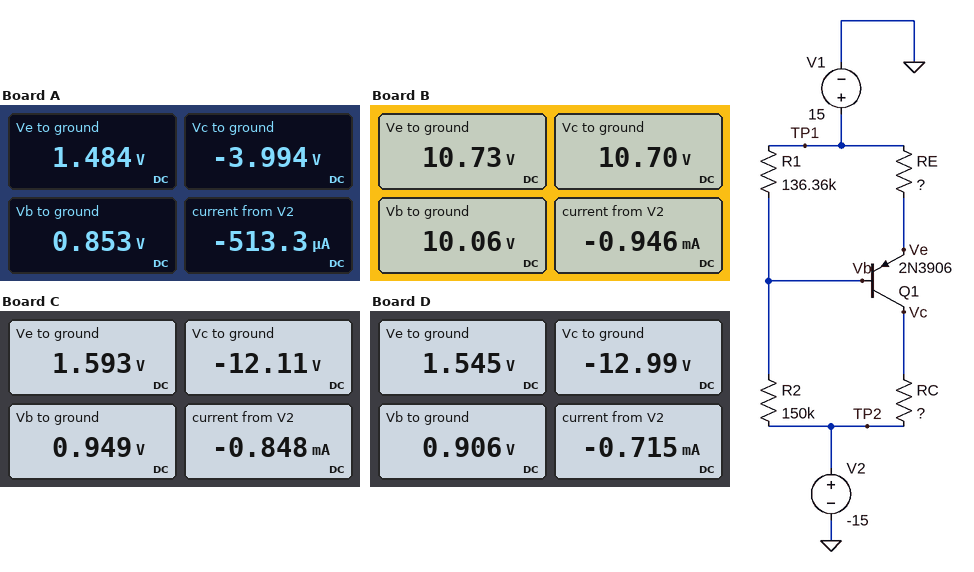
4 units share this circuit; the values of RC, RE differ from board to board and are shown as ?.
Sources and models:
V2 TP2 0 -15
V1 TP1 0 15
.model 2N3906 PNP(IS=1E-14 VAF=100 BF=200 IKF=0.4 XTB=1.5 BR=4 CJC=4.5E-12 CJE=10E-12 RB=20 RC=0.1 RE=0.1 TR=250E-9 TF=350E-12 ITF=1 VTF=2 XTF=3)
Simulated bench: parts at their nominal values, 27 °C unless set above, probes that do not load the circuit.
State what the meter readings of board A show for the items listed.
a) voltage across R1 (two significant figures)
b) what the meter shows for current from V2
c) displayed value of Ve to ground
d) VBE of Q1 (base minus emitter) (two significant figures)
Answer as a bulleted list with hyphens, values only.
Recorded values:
- 14 V
- -513.3 µA
- 1.484 V
- -630 mV
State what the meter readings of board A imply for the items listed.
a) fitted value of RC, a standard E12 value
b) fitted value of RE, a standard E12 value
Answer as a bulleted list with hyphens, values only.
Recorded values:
- 27 kΩ
- 33 kΩ
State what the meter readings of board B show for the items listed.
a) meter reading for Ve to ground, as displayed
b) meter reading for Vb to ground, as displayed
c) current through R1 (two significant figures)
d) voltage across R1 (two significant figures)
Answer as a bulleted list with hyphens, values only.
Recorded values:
- 10.73 V
- 10.06 V
- 36 µA
- 4.9 V
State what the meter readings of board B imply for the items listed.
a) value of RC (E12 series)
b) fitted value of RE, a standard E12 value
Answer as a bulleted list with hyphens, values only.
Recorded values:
- 33 kΩ
- 4.7 kΩ
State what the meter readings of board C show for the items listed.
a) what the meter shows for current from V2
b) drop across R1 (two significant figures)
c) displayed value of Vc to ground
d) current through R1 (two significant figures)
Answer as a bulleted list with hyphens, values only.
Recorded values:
- -0.848 mA
- 14 V
- -12.11 V
- 100 µA
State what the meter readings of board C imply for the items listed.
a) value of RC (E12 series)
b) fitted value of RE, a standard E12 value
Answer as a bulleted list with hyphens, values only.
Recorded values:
- 3.9 kΩ
- 18 kΩ
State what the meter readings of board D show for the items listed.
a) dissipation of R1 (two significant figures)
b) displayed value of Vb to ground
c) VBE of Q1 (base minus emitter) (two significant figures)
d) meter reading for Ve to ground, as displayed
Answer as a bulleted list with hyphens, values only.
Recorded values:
- 1.5 mW
- 0.906 V
- -640 mV
- 1.545 V
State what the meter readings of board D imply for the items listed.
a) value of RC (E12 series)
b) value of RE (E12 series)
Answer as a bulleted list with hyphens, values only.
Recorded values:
- 3.3 kΩ
- 22 kΩ
